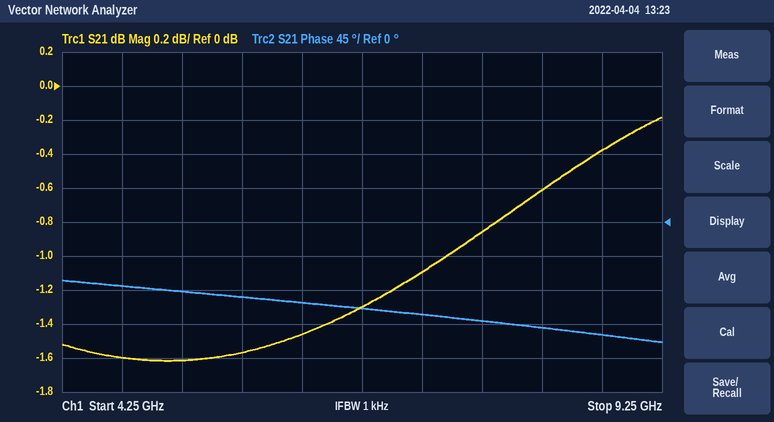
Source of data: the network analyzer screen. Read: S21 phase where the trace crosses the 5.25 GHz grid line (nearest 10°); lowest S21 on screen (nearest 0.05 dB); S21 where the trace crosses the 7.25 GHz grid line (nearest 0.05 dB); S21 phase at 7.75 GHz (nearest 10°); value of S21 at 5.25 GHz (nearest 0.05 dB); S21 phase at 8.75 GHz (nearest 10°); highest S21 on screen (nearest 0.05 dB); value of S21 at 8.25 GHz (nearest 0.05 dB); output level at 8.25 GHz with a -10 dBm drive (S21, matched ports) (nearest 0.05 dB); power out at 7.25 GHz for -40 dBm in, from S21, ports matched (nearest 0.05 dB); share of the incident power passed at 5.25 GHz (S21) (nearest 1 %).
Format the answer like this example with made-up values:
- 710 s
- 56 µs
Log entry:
- -90°
- -1.60 dB
- -1.10 dB
- -130°
- -1.60 dB
- -150°
- -0.20 dB
- -0.60 dB
- -10.60 dBm
- -41.10 dBm
- 69 %
